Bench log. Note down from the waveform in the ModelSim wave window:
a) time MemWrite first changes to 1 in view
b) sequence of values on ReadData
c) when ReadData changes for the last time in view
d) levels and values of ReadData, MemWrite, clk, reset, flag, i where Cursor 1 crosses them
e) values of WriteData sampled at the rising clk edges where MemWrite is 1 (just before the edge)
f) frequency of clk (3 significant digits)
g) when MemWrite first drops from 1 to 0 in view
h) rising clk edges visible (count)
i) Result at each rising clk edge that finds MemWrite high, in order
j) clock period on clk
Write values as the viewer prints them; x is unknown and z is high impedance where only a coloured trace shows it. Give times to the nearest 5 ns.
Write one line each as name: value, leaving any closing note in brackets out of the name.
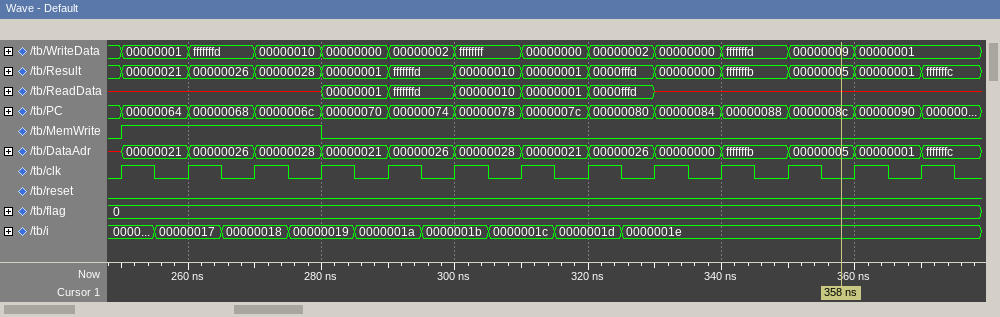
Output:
time MemWrite first changes to 1 in view: 250 ns
sequence of values on ReadData: x, 00000001, fffffffd, 00000010, 00000001, 0000fffd, x
when ReadData changes for the last time in view: 330 ns
levels and values of ReadData, MemWrite, clk, reset, flag, i where Cursor 1 crosses them: ReadData=x, MemWrite=0, clk=0, reset=0, flag=0, i=0000001e
values of WriteData sampled at the rising clk edges where MemWrite is 1: 00000001, fffffffd, 00000010
frequency of clk: 100 MHz
when MemWrite first drops from 1 to 0 in view: 280 ns
rising clk edges visible: 13
Result at each rising clk edge that finds MemWrite high, in order: 00000021, 00000026, 00000028
clock period on clk: 10 ns
